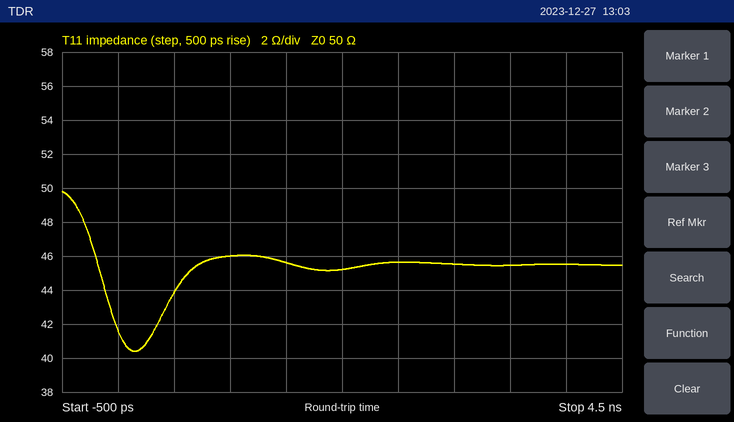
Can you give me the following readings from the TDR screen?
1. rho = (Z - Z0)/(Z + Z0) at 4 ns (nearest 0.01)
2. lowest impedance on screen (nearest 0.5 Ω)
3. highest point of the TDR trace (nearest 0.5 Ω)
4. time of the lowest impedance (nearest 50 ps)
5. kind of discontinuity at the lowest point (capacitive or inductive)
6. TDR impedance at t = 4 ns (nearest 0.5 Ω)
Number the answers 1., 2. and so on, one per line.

1. -0.05
2. 40.5 Ω
3. 50.0 Ω
4. 150 ps
5. capacitive
6. 45.5 Ω
